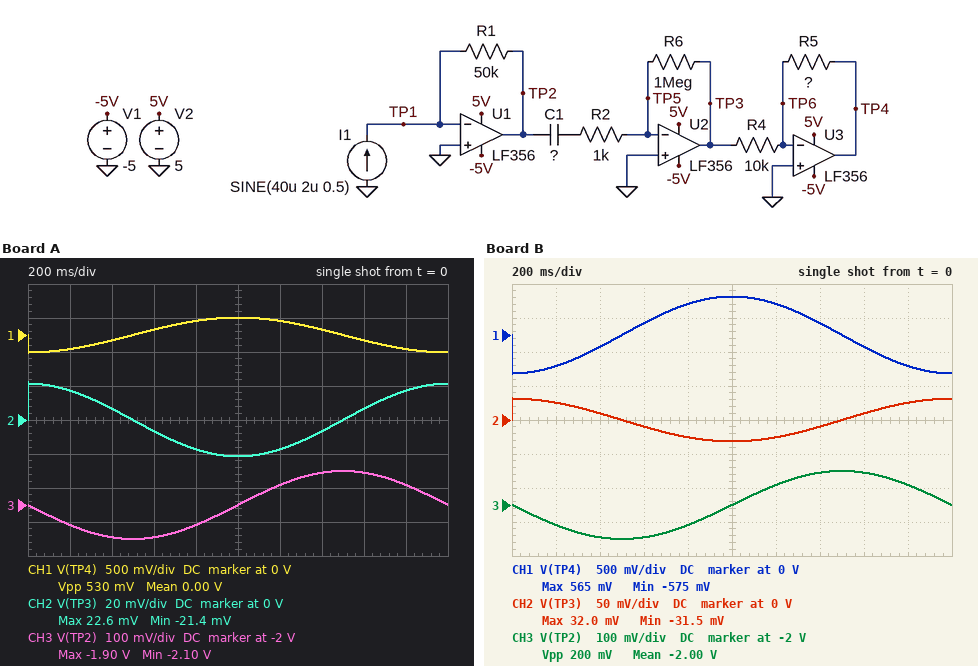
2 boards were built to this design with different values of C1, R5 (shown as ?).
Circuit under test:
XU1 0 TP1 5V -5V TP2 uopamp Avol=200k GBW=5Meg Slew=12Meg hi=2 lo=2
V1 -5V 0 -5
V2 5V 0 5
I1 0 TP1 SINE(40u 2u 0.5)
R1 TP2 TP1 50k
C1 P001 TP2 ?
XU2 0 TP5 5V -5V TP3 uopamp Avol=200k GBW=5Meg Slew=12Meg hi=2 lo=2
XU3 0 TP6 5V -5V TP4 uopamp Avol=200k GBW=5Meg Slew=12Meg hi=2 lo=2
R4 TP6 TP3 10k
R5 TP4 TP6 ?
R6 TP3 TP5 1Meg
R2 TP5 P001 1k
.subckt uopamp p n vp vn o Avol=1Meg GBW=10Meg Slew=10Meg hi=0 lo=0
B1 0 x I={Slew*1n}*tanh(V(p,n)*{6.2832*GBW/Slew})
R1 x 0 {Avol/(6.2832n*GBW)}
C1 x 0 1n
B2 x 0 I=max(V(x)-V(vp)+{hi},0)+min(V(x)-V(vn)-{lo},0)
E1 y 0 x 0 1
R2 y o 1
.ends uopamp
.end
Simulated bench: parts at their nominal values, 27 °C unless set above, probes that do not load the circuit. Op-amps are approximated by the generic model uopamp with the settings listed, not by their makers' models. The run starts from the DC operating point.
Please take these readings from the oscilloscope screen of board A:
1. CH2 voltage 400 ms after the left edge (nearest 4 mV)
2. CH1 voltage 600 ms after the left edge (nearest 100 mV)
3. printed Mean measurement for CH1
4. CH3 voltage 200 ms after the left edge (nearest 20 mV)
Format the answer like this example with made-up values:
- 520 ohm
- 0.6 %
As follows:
- 8 mV
- 100 mV
- 0.00 V
- -2.06 V
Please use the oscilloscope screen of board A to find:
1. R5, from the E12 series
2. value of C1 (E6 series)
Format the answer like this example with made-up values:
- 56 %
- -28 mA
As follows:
- 120 kΩ
- 68 nF
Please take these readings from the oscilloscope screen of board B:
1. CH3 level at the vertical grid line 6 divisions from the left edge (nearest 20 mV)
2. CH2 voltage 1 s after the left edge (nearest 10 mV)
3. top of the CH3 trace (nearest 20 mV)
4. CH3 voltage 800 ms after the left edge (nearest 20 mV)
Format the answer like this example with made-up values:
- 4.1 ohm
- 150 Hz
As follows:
- -1.94 V
- -30 mV
- -1.90 V
- -2.06 V
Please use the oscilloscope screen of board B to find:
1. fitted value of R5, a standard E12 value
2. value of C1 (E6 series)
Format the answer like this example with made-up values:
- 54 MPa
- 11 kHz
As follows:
- 180 kΩ
- 100 nF
